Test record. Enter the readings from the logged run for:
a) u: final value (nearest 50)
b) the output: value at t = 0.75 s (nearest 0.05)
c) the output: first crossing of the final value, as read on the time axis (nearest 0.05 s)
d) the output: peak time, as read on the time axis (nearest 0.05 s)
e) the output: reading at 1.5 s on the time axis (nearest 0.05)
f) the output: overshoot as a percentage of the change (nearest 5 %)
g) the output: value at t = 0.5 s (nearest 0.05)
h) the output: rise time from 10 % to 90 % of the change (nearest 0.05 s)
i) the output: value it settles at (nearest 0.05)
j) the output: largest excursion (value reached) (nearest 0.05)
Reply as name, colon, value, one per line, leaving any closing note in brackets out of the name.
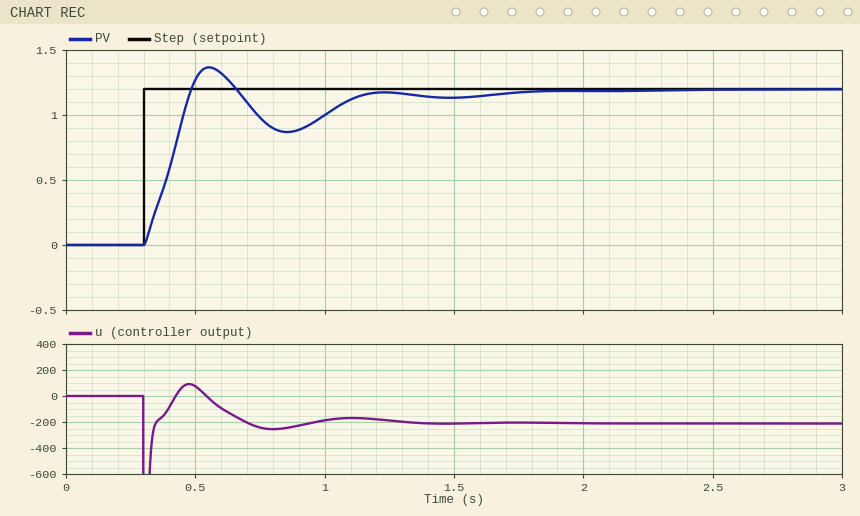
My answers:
u: final value: -200
the output: value at t = 0.75 s: 1.00
the output: first crossing of the final value, as read on the time axis: 0.50 s
the output: peak time, as read on the time axis: 0.55 s
the output: reading at 1.5 s on the time axis: 1.15
the output: overshoot as a percentage of the change: 15 %
the output: value at t = 0.5 s: 1.25
the output: rise time from 10 % to 90 % of the change: 0.15 s
the output: value it settles at: 1.20
the output: largest excursion (value reached): 1.35
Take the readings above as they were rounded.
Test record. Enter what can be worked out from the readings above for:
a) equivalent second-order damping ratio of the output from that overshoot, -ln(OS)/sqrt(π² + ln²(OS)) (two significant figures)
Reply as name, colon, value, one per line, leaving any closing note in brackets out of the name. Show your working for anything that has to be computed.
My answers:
equivalent second-order damping ratio of the output from that overshoot, -ln(OS)/sqrt(π² + ln²(OS)): ln(0.15) = -1.897; 1.897 / sqrt(9.870 + 3.599) = 0.52
